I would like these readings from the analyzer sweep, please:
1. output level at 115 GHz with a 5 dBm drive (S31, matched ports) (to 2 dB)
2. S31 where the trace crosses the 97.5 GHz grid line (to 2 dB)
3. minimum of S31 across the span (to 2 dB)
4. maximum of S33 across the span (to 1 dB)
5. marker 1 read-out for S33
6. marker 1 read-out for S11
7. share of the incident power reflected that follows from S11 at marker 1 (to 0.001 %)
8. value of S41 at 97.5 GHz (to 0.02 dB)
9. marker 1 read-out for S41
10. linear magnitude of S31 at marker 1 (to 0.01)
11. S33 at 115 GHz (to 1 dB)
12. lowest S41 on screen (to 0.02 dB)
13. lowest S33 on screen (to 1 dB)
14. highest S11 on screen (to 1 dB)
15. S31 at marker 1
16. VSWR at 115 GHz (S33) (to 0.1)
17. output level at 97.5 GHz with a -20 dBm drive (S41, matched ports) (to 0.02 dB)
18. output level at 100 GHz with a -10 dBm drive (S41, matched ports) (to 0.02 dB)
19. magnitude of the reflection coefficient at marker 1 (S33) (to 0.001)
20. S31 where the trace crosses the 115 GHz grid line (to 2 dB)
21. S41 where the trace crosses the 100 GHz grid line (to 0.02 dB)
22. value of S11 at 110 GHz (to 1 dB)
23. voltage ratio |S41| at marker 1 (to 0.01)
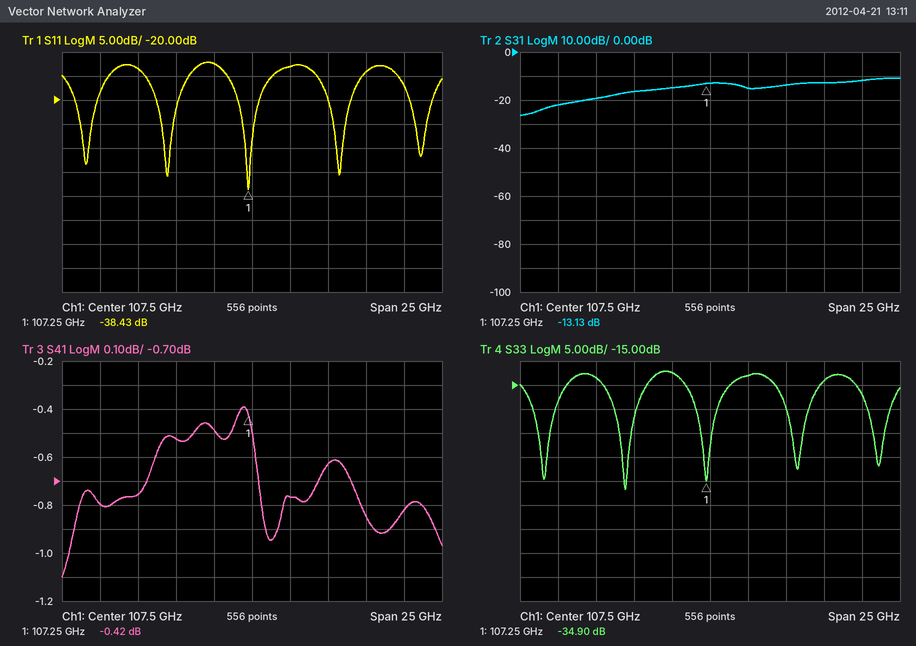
-8 dBm
-22 dB
-26 dB
-12 dB
-34.90 dB
-38.43 dB
0.014 %
-0.80 dB
-0.42 dB
0.22
-14 dB
-1.10 dB
-37 dB
-12 dB
-13.13 dB
1.5
-20.80 dBm
-10.76 dBm
0.018
-12 dB
-0.76 dB
-13 dB
0.95
